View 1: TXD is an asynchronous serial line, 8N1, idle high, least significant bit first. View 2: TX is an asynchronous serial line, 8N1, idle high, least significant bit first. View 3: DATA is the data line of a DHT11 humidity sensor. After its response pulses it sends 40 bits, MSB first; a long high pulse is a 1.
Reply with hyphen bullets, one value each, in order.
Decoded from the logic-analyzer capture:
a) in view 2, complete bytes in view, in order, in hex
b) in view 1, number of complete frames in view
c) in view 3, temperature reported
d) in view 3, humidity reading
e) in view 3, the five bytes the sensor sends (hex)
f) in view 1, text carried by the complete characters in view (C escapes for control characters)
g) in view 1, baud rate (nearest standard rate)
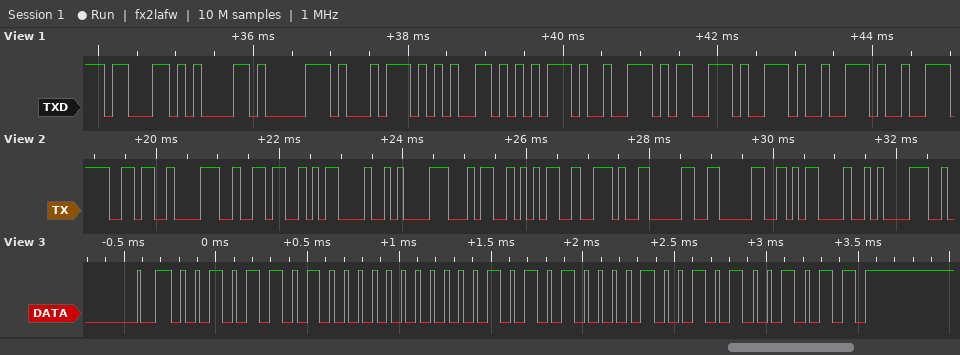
- 0x36 0x38 0x36 0x0D 0x0A 0x34 0x35 0x2E 0x30 0x30 0x0D 0x0A
- 10
- 21.9 °C
- 45 %
- 2D 00 15 09 4B
- "capteurs.."
- 9600 baud
